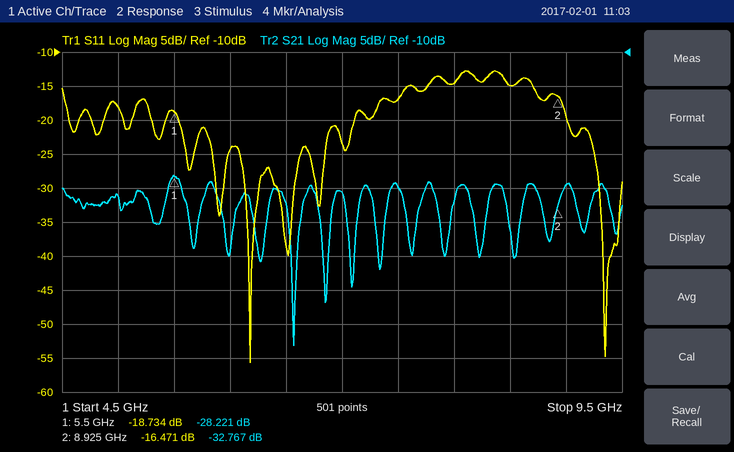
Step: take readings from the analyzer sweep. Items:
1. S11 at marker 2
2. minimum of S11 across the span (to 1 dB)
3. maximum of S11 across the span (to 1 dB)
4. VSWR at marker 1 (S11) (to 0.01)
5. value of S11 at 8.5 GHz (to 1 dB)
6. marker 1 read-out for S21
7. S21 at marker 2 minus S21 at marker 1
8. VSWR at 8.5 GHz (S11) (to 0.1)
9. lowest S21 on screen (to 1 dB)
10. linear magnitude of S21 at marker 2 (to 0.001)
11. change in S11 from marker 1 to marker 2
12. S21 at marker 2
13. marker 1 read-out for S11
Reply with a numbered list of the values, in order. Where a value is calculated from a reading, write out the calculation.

1. -16.471 dB
2. -56 dB
3. -13 dB
4. (1 + 0.1157)/(1 − 0.1157) ≈ 1.26
5. -15 dB
6. -28.221 dB
7. -32.767 − (-28.221) = -4.546 dB
8. |Γ| = 10^(-15/20) = 0.1778; VSWR = (1 + 0.1778)/(1 − 0.1778) ≈ 1.4
9. -53 dB
10. 10^(-32.767/20) ≈ 0.023
11. -16.471 − (-18.734) = 2.263 dB
12. -32.767 dB
13. -18.734 dB
